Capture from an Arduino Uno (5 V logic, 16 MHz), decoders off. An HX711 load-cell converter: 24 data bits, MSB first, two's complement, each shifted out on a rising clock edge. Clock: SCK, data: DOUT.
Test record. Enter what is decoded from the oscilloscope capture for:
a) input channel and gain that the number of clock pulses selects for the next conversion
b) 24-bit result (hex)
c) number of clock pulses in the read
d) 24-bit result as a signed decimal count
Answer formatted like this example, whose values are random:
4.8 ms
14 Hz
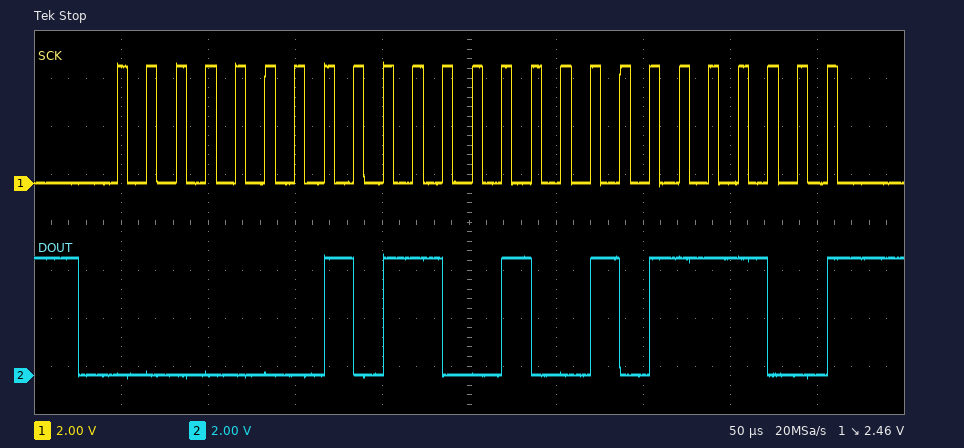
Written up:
channel A, gain 128
0x0164BC
25
91324
